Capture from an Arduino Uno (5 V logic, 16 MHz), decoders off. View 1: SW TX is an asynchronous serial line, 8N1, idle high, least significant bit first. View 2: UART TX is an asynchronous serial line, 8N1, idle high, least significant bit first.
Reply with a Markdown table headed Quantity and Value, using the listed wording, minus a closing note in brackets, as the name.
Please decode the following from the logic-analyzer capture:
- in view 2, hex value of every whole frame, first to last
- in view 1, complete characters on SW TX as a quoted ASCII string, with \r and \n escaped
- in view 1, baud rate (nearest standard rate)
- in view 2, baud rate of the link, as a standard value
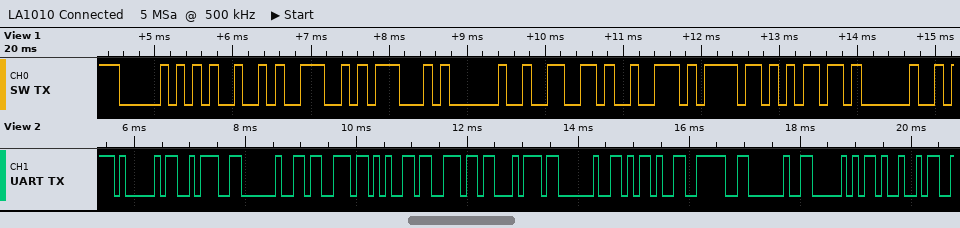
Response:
| Quantity | Value |
|---|---|
| in view 2, hex value of every whole frame, first to last | 0x41 0x3A 0x20 0x73 0x65 0x6E 0x74 0x20 0x2D 0x3E 0x20 0x50 0x49 |
| in view 1, complete characters on SW TX as a quoted ASCII string, with \r and \n escaped | "PING from " |
| in view 1, baud rate | 9600 baud |
| in view 2, baud rate of the link, as a standard value | 9600 baud |
